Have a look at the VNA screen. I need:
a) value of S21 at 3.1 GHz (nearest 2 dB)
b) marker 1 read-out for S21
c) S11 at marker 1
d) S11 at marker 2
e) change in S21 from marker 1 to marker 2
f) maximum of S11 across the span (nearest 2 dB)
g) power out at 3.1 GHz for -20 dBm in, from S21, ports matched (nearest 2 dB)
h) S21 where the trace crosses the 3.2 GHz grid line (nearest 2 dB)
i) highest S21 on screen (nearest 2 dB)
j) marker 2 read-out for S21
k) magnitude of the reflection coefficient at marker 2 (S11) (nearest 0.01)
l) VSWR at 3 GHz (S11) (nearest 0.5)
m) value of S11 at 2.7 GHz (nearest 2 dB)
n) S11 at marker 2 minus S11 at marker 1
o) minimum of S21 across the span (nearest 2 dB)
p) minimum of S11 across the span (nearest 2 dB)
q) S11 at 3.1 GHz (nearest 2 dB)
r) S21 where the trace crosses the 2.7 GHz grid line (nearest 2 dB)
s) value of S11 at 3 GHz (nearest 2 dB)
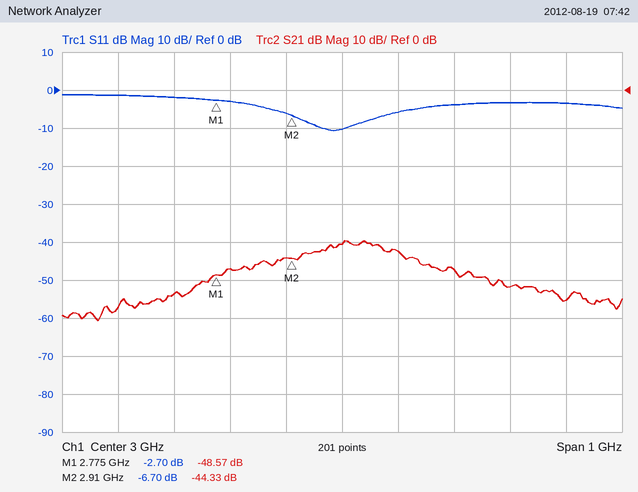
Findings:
-42 dB
-48.57 dB
-2.70 dB
-6.70 dB
4.24 dB
-2 dB
-62 dBm
-48 dB
-40 dB
-44.33 dB
0.46
2.0
-2 dB
-4.00 dB
-60 dB
-10 dB
-6 dB
-54 dB
-10 dB
